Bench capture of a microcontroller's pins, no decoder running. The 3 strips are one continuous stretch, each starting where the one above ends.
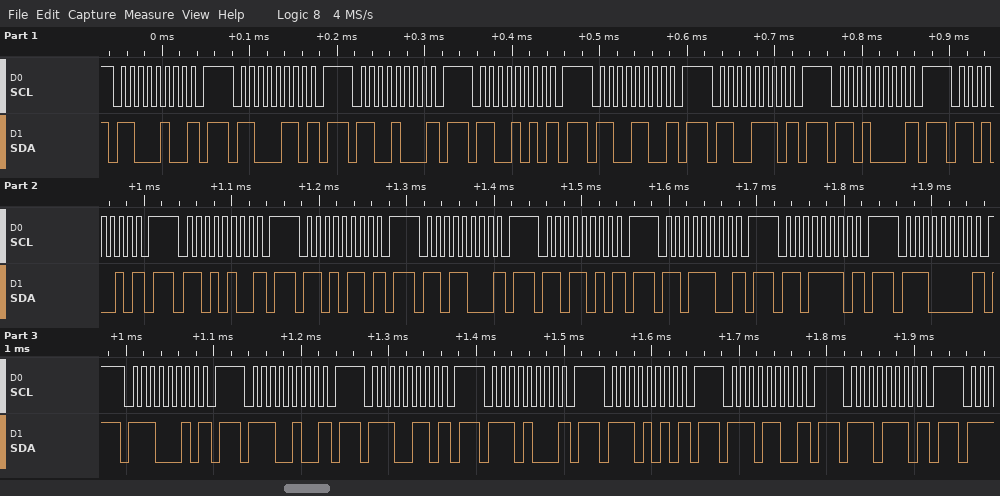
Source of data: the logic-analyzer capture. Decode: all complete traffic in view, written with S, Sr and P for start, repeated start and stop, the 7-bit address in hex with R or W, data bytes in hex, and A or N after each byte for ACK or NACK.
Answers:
S 62W N P S 63W N P S 64W N P S 65W N P S 66W N P S 67W N P S 68W N P S 69W N P S 6AW N P S 6BW N P S 6CW N P S 6DW N P S 6EW N P S 6FW N P S 70W N P S 71W N P S 72W N P S 73W N P S 74W N P S 75W N P S 76W N P S 77W N P
